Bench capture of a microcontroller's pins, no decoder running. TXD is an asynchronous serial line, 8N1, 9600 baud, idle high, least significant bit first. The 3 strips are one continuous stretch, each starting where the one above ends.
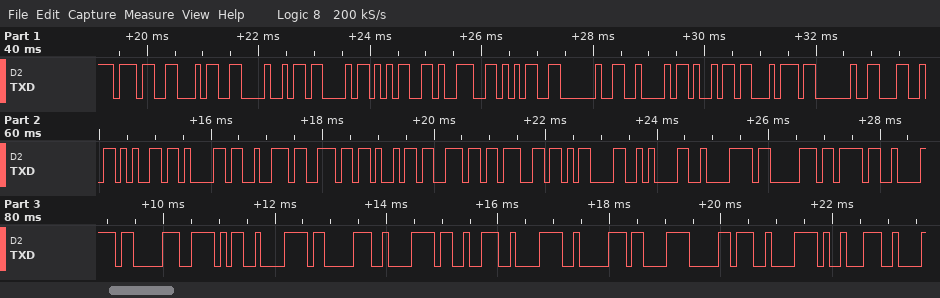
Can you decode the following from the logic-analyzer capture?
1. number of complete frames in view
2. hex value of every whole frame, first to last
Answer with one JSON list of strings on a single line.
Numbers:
["38", "37 34 48 43 35 39 35 20 42 69 74 20 4C 65 61 72 6E 69 6E 67 0D 0A C2 83 7B C2 83 5E C2 83 C2 93 C2 82 C3 B0 C2 89"]
